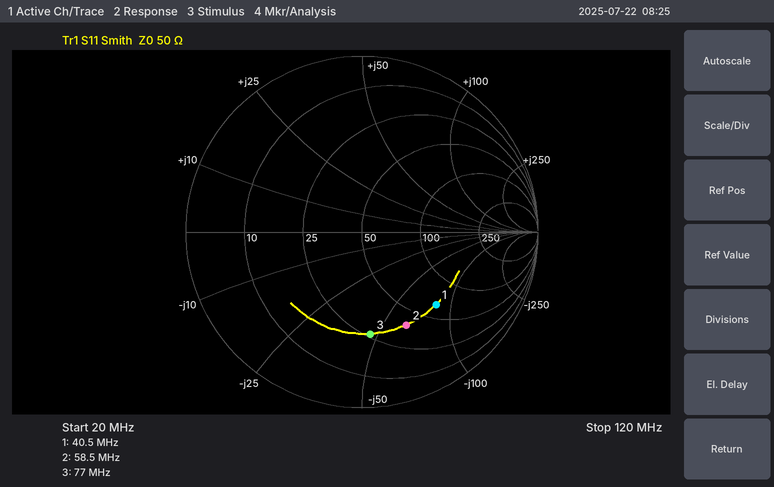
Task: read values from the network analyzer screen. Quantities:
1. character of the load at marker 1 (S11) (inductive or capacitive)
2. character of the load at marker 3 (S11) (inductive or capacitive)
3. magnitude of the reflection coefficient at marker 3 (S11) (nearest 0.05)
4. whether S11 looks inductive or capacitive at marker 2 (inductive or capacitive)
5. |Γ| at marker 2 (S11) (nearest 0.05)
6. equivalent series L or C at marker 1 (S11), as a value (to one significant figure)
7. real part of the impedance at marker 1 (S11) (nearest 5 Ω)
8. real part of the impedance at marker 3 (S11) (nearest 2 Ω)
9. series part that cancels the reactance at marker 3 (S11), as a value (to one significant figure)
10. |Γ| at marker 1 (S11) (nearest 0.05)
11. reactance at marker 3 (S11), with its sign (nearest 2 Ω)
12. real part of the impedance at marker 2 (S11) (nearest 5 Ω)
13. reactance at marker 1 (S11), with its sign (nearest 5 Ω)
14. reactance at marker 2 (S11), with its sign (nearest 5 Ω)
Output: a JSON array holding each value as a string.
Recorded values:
["capacitive", "capacitive", "0.60", "capacitive", "0.60", "50 pF", "65 Ω", "26 Ω", "100 nH", "0.60", "-46 Ω", "40 Ω", "-80 Ω", "-65 Ω"]
